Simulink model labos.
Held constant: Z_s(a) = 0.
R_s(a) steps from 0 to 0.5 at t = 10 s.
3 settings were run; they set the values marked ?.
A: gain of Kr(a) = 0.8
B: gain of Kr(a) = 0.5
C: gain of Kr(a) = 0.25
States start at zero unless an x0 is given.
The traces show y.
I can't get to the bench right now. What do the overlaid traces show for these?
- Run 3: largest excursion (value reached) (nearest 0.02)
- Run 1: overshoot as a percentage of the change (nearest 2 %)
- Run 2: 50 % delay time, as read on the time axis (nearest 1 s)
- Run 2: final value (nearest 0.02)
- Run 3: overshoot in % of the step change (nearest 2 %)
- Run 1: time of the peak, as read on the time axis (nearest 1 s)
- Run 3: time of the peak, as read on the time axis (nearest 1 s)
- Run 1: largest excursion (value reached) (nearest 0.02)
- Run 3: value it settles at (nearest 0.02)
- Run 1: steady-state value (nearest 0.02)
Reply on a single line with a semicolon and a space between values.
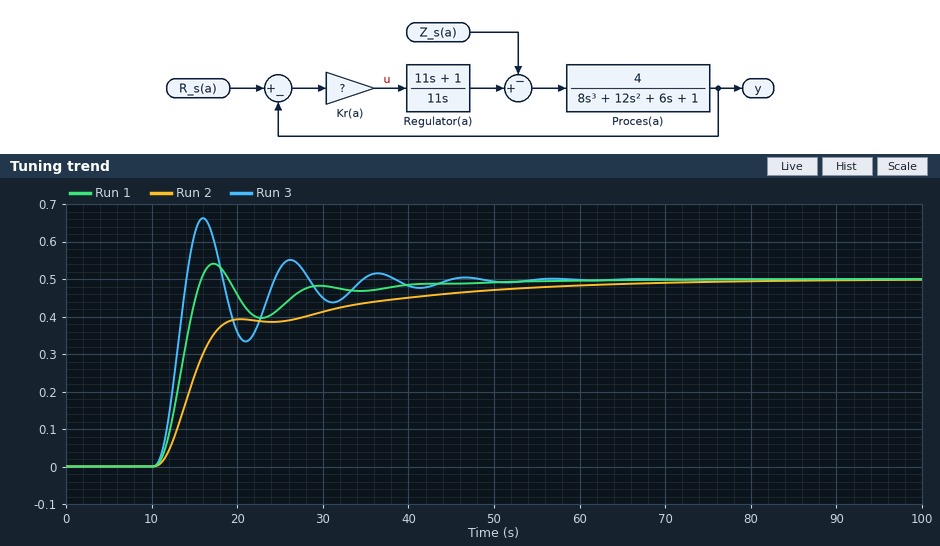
0.66; 8 %; 15 s; 0.50; 32 %; 17 s; 16 s; 0.54; 0.50; 0.50
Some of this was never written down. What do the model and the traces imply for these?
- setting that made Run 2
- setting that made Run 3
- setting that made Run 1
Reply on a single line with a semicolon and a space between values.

C; A; B
